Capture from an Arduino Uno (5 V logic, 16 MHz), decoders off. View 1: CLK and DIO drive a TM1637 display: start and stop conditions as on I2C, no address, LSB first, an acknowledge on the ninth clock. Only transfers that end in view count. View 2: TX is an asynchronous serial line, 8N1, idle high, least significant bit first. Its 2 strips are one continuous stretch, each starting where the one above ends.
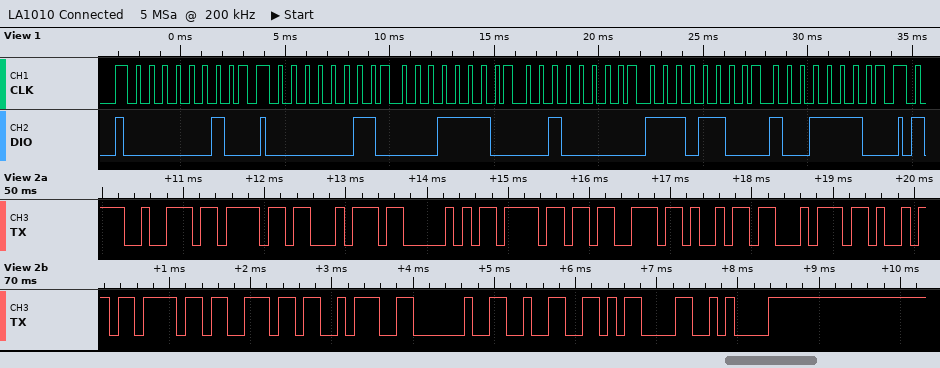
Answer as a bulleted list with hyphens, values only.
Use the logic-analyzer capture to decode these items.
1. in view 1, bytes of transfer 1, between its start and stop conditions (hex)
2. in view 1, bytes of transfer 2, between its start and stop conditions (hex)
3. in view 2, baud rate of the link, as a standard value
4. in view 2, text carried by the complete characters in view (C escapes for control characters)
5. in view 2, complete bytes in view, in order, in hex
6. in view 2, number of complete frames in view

- 40
- C0 78 04 37 79
- 9600 baud
- "rotPosition: 2\r\n"
- 72 6F 74 50 6F 73 69 74 69 6F 6E 3A 20 32 0D 0A
- 16
